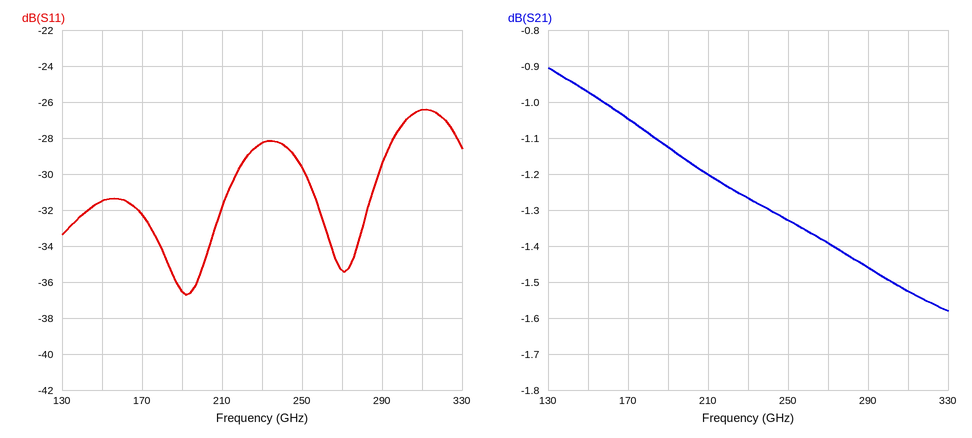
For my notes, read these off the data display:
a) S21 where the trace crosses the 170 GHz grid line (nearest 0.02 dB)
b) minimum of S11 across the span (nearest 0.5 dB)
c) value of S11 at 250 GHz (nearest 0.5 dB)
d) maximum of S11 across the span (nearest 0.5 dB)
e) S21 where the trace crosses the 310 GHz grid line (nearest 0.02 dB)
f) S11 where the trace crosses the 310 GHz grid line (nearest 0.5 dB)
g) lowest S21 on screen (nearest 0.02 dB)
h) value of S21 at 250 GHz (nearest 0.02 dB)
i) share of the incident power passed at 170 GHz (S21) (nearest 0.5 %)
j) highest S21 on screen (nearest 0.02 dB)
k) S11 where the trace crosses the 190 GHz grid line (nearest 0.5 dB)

-1.04 dB
-36.5 dB
-29.5 dB
-26.5 dB
-1.52 dB
-26.5 dB
-1.58 dB
-1.32 dB
78.5 %
-0.90 dB
-36.5 dB
